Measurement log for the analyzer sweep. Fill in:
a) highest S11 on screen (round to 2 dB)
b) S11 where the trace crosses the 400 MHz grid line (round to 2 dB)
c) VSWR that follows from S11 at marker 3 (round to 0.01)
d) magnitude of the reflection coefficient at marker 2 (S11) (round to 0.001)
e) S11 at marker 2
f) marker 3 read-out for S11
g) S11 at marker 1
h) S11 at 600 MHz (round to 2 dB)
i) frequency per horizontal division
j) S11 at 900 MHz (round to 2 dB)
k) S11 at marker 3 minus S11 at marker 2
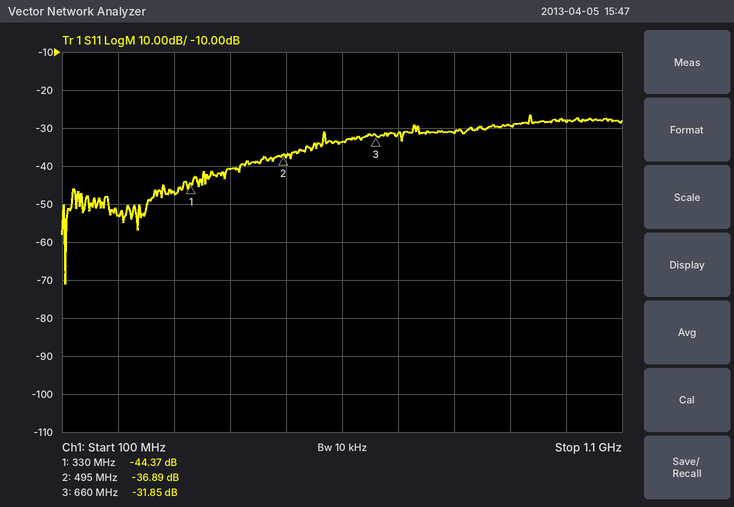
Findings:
-26 dB
-40 dB
1.05
0.014
-36.89 dB
-31.85 dB
-44.37 dB
-34 dB
100 MHz
-30 dB
5.04 dB
